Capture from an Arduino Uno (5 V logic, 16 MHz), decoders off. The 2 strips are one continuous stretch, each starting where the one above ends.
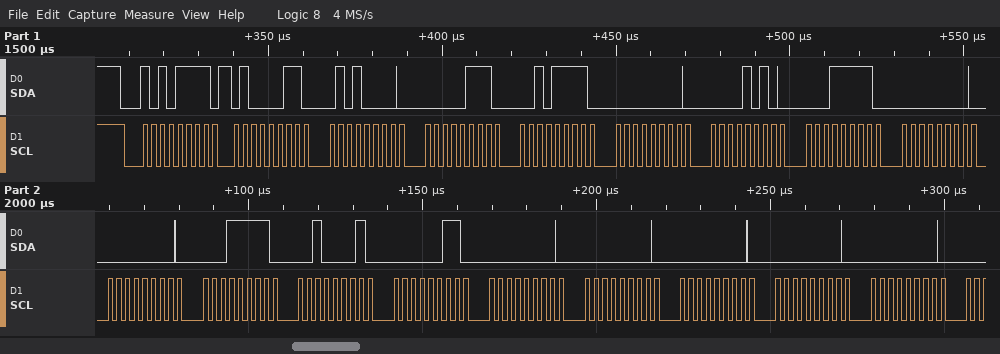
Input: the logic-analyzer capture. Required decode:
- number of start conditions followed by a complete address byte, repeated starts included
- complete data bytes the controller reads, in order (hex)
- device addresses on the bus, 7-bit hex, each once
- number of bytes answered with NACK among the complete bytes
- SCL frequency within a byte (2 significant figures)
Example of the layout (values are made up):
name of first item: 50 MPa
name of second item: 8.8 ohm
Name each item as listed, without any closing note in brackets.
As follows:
number of start conditions followed by a complete address byte, repeated starts included: 1
complete data bytes the controller reads, in order: 43 50 07 2F 00 0A 1F 00 00 1F 21 03 00 00 00 00 00
device addresses on the bus, 7-bit hex, each once: 0x57
number of bytes answered with NACK among the complete bytes: 0
SCL frequency within a byte: 400 kHz
